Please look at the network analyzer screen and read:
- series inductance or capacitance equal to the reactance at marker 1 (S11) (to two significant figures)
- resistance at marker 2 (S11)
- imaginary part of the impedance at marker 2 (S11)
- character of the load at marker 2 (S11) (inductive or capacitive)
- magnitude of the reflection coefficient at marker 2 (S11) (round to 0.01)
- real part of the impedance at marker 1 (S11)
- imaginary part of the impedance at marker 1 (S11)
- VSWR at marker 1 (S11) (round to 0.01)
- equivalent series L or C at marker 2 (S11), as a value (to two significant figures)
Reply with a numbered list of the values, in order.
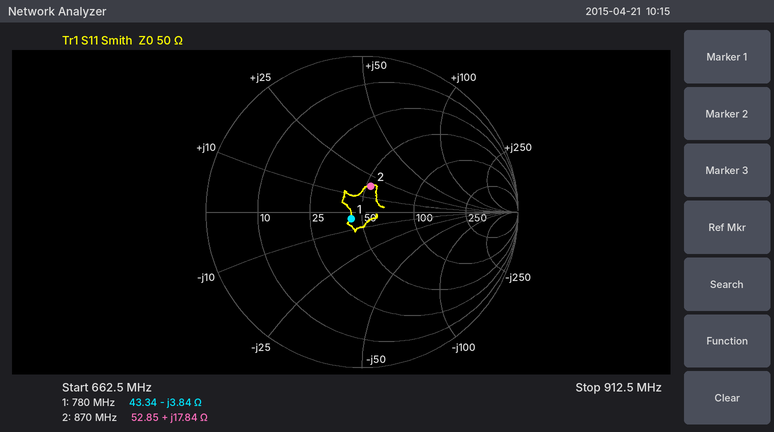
1. 53 pF
2. 52.85 Ω
3. +17.84 Ω
4. inductive
5. 0.17
6. 43.34 Ω
7. -3.84 Ω
8. 1.18
9. 3.3 nH
